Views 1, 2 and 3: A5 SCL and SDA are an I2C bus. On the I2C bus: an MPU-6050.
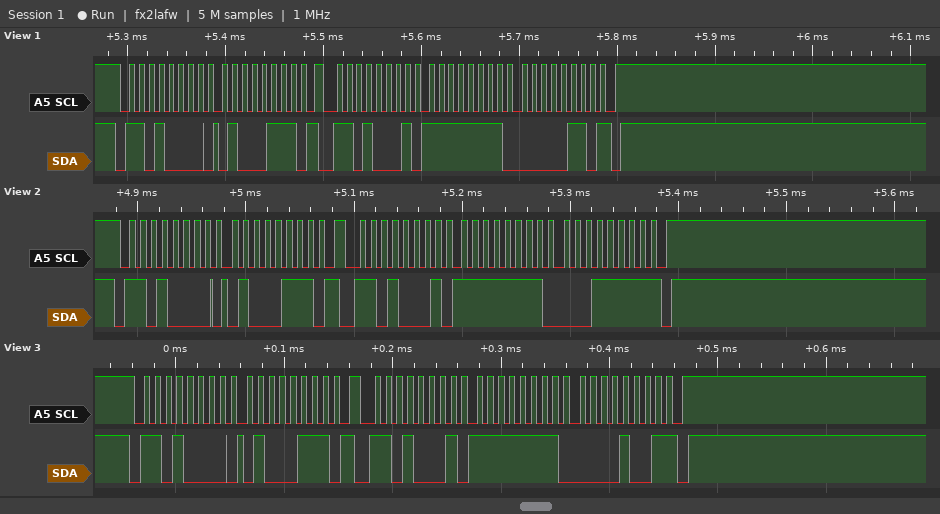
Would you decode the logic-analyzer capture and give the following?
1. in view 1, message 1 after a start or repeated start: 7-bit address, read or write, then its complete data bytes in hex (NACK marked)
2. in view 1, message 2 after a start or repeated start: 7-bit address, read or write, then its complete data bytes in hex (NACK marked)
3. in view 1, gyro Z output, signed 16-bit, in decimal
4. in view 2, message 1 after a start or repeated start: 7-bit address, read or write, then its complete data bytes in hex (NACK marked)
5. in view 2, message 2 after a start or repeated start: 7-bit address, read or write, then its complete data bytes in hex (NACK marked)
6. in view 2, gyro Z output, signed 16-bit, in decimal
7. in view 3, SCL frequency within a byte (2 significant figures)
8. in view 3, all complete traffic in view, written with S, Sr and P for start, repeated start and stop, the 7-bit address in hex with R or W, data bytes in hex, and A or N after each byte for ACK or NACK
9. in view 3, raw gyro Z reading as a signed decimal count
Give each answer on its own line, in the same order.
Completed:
0x68 write: 47
0x68 read: FF 06 NACK
-250
0x68 write: 47
0x68 read: FF 1F NACK
-225
100 kHz
S 68W A 47 A Sr 68R A FF A 09 N P
-247
